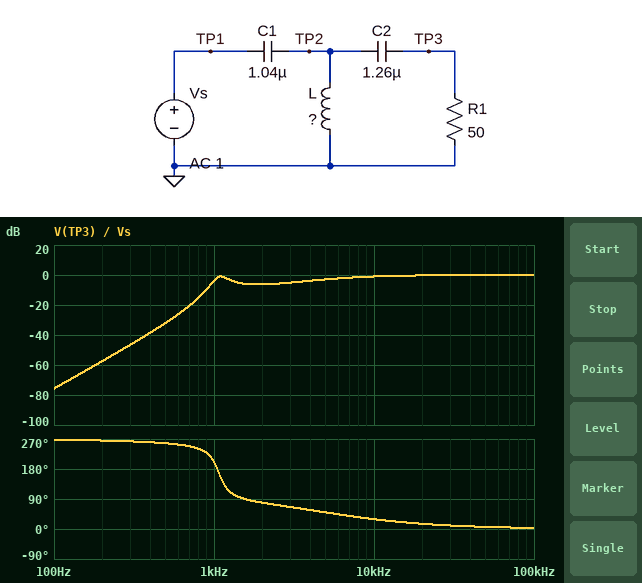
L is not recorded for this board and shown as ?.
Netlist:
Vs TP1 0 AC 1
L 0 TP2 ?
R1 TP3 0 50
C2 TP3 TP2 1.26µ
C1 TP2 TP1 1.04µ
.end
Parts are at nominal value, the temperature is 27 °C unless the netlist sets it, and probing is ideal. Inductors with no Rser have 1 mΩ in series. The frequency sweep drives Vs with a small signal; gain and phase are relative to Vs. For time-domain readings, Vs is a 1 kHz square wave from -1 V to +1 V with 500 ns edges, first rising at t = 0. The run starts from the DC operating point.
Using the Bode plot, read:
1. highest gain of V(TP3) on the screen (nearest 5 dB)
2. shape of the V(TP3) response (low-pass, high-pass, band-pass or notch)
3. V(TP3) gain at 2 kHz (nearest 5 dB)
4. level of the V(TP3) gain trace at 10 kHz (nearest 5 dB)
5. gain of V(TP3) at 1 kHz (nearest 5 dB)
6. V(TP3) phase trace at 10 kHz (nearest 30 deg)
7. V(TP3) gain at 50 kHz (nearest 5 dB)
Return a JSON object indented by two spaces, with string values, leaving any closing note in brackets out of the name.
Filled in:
{
  "highest gain of V(TP3) on the screen": "0 dB",
  "shape of the V(TP3) response": "high-pass",
  "V(TP3) gain at 2 kHz": "-5 dB",
  "level of the V(TP3) gain trace at 10 kHz": "0 dB",
  "gain of V(TP3) at 1 kHz": "-5 dB",
  "V(TP3) phase trace at 10 kHz": "30 deg",
  "V(TP3) gain at 50 kHz": "0 dB"
}
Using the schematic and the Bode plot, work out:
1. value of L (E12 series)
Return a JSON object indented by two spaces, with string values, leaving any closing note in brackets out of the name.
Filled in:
{
  "value of L": "10 mH"
}
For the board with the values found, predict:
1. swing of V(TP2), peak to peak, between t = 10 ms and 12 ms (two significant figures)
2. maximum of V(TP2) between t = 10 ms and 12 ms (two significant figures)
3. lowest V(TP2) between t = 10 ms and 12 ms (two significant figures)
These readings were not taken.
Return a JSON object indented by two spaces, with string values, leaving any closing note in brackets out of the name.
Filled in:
{
  "swing of V(TP2), peak to peak, between t = 10 ms and 12 ms": "6.2 V",
  "maximum of V(TP2) between t = 10 ms and 12 ms": "3.1 V",
  "lowest V(TP2) between t = 10 ms and 12 ms": "-3.1 V"
}
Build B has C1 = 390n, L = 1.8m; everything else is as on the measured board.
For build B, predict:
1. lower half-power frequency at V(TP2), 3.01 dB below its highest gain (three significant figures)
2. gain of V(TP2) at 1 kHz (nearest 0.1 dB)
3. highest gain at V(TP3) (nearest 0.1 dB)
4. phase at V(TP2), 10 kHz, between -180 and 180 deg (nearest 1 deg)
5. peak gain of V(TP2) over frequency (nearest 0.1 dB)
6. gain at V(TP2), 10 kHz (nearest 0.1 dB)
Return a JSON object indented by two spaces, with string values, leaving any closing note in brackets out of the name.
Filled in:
{
  "lower half-power frequency at V(TP2), 3.01 dB below its highest gain": "4.31 kHz",
  "gain of V(TP2) at 1 kHz": "-30.2 dB",
  "highest gain at V(TP3)": "0 dB",
  "phase at V(TP2), 10 kHz, between -180 and 180 deg": "43 deg",
  "peak gain of V(TP2) over frequency": "0 dB",
  "gain at V(TP2), 10 kHz": "-1.1 dB"
}
